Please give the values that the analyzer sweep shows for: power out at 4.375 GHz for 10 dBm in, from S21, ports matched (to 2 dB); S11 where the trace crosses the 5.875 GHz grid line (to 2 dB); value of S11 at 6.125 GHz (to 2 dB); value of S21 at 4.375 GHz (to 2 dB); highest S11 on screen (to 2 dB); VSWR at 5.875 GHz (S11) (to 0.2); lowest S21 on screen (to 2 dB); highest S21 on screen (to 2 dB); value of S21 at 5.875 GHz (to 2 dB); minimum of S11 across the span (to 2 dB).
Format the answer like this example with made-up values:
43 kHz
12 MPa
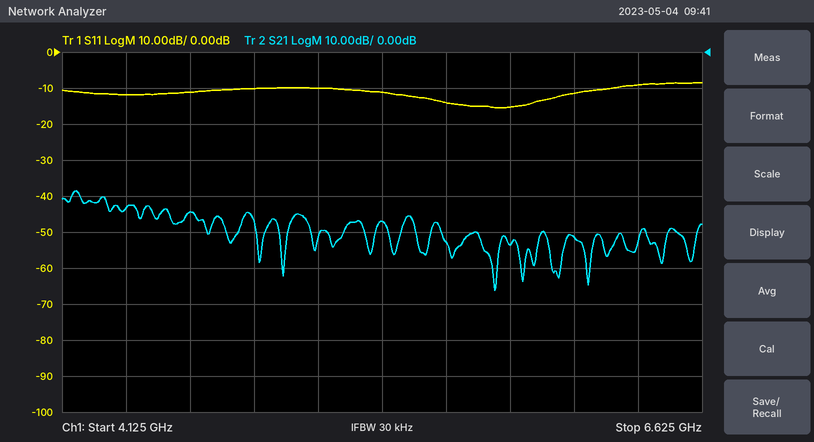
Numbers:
-34 dBm
-16 dB
-12 dB
-44 dB
-8 dB
1.4
-66 dB
-38 dB
-54 dB
-16 dB
